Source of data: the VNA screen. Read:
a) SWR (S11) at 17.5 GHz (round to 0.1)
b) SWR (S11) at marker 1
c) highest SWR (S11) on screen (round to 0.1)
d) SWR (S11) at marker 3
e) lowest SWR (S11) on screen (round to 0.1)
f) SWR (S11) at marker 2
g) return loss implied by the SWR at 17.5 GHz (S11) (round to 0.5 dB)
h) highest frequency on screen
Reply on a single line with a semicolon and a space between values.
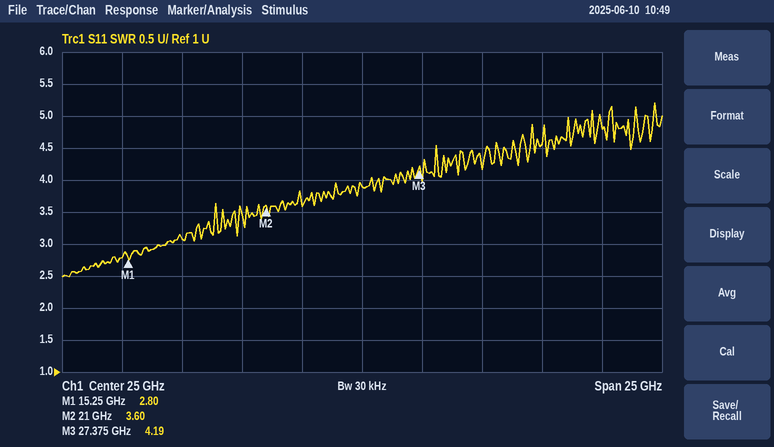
3.1; 2.80; 5.2; 4.19; 2.5; 3.60; 6.0 dB; 37.5 GHz
